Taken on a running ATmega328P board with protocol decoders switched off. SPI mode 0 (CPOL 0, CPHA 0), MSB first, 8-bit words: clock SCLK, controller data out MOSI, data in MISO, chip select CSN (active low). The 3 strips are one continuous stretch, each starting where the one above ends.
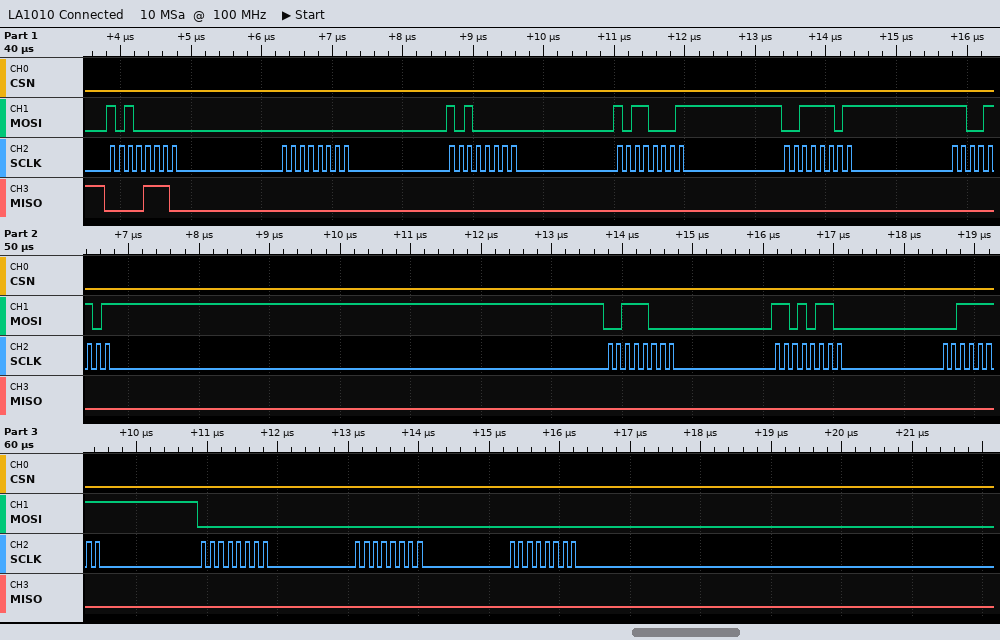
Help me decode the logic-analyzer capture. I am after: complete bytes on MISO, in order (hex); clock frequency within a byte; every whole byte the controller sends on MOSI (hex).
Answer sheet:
0E 00 00 00 00 00 00 00 00 00 00 00
8 MHz
A0 00 A0 B1 3D CD 38 D6 3F 00 00 00
